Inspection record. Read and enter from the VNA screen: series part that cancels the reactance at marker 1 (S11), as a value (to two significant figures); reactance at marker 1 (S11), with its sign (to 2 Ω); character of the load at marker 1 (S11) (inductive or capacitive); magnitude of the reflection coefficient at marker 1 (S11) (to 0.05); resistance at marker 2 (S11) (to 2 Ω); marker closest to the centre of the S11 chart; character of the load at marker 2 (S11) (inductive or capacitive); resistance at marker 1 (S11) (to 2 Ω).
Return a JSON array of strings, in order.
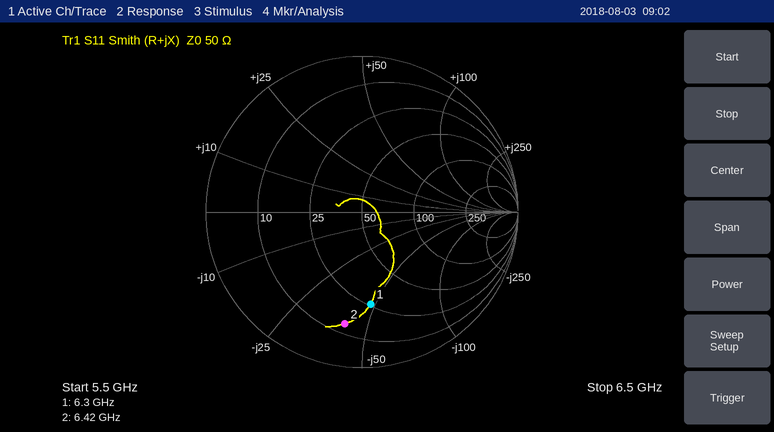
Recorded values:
["1.2 nH", "-48 Ω", "capacitive", "0.60", "14 Ω", "marker 1", "capacitive", "26 Ω"]
